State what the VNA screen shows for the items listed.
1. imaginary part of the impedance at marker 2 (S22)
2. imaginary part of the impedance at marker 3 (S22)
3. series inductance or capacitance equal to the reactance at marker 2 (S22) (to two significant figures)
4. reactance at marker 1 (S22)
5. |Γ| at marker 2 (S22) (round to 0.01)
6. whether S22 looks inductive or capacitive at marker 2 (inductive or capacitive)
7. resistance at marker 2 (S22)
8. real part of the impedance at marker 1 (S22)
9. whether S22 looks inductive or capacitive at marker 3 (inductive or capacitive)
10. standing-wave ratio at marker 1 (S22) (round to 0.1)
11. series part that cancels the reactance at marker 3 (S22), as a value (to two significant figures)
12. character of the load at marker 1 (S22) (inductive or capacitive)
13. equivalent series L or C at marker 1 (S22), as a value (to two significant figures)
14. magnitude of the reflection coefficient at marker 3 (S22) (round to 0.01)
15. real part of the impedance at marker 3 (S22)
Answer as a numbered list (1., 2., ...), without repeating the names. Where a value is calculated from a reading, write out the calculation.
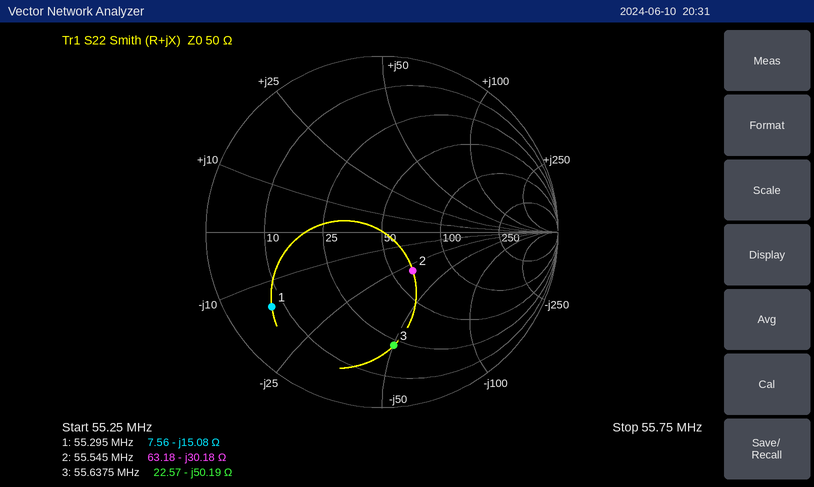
1. -30.18 Ω
2. -50.19 Ω
3. C = 1/(2π × 55.545 MHz × 30.18 Ω) ≈ 95 pF
4. -15.08 Ω
5. 0.28
6. capacitive
7. 63.18 Ω
8. 7.56 Ω
9. capacitive
10. 7.2
11. L = 50.19 Ω/(2π × 55.6375 MHz) ≈ 144 nH, so 140 nH to two significant figures
12. capacitive
13. C = 1/(2π × 55.295 MHz × 15.08 Ω) ≈ 191 pF, so 190 pF to two significant figures
14. 0.65
15. 22.57 Ω
